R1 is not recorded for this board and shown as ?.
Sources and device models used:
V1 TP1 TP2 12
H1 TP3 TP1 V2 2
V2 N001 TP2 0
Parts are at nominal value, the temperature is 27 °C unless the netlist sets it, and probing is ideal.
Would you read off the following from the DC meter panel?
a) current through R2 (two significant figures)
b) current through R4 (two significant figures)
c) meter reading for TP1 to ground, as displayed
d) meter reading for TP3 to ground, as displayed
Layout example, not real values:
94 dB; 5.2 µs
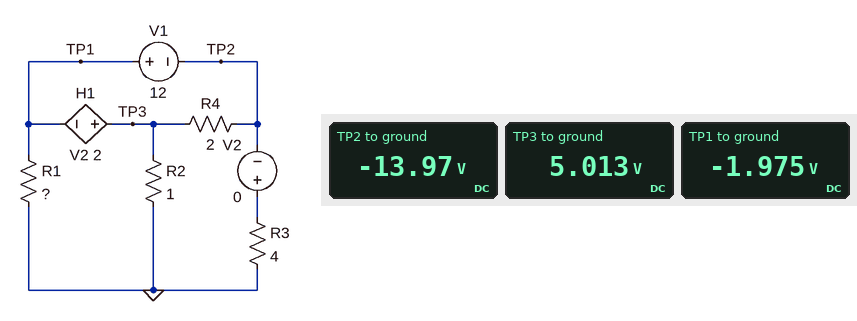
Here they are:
5.0 A; 9.5 A; -1.975 V; 5.013 V
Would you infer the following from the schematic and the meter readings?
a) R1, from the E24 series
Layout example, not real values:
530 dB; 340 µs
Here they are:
1.3 Ω
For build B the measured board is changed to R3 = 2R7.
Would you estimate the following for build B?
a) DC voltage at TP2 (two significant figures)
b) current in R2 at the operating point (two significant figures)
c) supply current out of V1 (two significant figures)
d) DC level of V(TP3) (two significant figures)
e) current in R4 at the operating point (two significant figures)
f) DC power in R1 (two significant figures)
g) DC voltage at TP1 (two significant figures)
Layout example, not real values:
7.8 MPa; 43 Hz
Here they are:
-15 V; 8.1 A; 17 A; 8.1 V; 12 A; 7.8 W; -3.2 V
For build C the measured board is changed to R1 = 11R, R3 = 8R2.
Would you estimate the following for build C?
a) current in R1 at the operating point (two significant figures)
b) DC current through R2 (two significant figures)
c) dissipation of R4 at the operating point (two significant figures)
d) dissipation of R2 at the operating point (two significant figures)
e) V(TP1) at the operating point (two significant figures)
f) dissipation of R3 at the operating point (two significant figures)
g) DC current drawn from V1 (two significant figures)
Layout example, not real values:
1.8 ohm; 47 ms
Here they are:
140 mA; 1.8 A; 120 W; 3.2 W; -1.5 V; 22 W; 9.3 A
